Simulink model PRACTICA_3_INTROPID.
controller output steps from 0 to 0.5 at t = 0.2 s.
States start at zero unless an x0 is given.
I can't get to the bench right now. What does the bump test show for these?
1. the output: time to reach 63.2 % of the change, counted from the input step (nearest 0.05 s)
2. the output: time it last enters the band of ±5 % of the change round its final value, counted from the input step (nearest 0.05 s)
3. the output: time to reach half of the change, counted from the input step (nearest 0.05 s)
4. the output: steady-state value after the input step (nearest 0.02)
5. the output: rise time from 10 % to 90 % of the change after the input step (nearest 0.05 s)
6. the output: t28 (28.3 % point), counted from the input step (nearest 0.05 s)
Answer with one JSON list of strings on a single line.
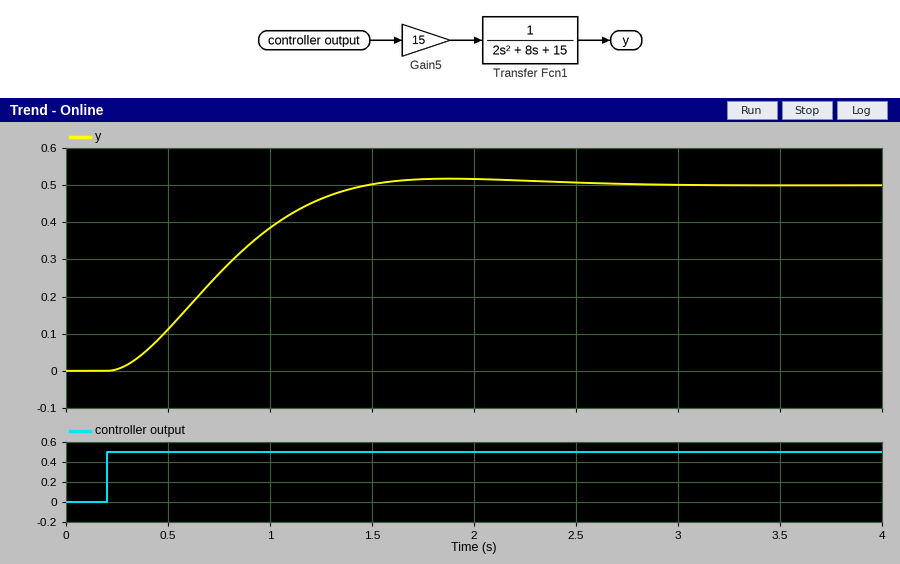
["0.65 s", "1.10 s", "0.55 s", "0.50", "0.80 s", "0.35 s"]
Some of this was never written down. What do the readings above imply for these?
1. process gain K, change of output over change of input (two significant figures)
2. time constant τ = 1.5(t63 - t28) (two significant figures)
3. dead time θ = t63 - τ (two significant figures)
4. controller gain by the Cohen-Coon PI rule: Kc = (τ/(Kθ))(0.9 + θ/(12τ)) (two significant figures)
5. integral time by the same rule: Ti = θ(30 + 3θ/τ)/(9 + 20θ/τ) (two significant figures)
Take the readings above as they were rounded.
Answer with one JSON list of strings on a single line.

["1.0", "0.45 s", "0.20 s", "2.1", "0.35 s"]
